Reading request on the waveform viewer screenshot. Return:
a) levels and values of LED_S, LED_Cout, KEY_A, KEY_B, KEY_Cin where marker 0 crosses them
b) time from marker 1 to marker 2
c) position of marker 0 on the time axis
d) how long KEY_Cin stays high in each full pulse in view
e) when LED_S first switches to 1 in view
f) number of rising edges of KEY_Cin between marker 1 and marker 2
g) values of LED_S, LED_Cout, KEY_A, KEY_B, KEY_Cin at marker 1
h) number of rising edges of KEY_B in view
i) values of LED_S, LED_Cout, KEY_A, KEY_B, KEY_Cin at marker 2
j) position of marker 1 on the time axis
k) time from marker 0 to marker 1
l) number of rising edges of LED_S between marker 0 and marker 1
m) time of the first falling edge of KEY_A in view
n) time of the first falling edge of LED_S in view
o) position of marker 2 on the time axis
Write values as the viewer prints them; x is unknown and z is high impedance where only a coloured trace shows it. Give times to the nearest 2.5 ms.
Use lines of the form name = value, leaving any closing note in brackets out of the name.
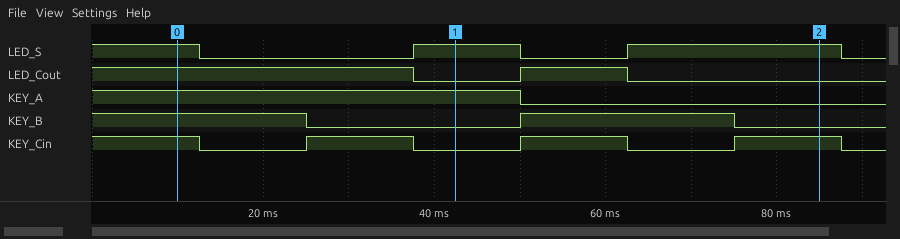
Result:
levels and values of LED_S, LED_Cout, KEY_A, KEY_B, KEY_Cin where marker 0 crosses them = LED_S=1, LED_Cout=1, KEY_A=1, KEY_B=1, KEY_Cin=1
time from marker 1 to marker 2 = 42.5 ms
position of marker 0 on the time axis = 10 ms
how long KEY_Cin stays high in each full pulse in view = 12.5 ms, 12.5 ms, 12.5 ms
when LED_S first switches to 1 in view = 37.5 ms
number of rising edges of KEY_Cin between marker 1 and marker 2 = 2
values of LED_S, LED_Cout, KEY_A, KEY_B, KEY_Cin at marker 1 = LED_S=1, LED_Cout=0, KEY_A=1, KEY_B=0, KEY_Cin=0
number of rising edges of KEY_B in view = 1
values of LED_S, LED_Cout, KEY_A, KEY_B, KEY_Cin at marker 2 = LED_S=1, LED_Cout=0, KEY_A=0, KEY_B=0, KEY_Cin=1
position of marker 1 on the time axis = 42.5 ms
time from marker 0 to marker 1 = 32.5 ms
number of rising edges of LED_S between marker 0 and marker 1 = 1
time of the first falling edge of KEY_A in view = 50 ms
time of the first falling edge of LED_S in view = 12.5 ms
position of marker 2 on the time axis = 85 ms
